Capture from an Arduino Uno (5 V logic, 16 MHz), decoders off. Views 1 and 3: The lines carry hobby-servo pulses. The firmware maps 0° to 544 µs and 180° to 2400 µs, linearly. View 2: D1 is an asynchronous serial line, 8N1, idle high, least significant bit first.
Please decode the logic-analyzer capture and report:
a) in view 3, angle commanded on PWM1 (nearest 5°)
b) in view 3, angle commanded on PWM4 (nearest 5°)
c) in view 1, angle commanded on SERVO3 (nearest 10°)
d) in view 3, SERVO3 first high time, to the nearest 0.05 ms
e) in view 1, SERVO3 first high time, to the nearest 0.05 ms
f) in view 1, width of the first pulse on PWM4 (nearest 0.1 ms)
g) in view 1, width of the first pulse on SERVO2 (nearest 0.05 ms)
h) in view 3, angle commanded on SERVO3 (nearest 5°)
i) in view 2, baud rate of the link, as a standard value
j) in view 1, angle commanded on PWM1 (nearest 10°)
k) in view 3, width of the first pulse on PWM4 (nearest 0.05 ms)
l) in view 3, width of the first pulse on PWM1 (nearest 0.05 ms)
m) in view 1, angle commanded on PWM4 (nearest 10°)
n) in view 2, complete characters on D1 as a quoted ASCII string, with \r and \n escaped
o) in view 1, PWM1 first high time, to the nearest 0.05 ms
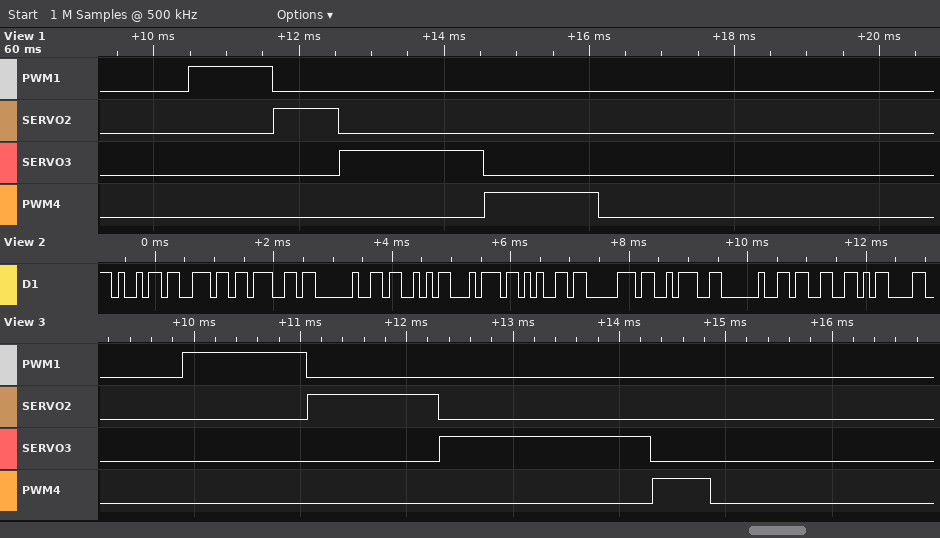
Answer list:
60°
0°
140°
2.00 ms
2.00 ms
1.6 ms
0.90 ms
140°
9600 baud
60°
0.55 ms
1.15 ms
100°
"ing Step: 3\r"
1.15 ms
